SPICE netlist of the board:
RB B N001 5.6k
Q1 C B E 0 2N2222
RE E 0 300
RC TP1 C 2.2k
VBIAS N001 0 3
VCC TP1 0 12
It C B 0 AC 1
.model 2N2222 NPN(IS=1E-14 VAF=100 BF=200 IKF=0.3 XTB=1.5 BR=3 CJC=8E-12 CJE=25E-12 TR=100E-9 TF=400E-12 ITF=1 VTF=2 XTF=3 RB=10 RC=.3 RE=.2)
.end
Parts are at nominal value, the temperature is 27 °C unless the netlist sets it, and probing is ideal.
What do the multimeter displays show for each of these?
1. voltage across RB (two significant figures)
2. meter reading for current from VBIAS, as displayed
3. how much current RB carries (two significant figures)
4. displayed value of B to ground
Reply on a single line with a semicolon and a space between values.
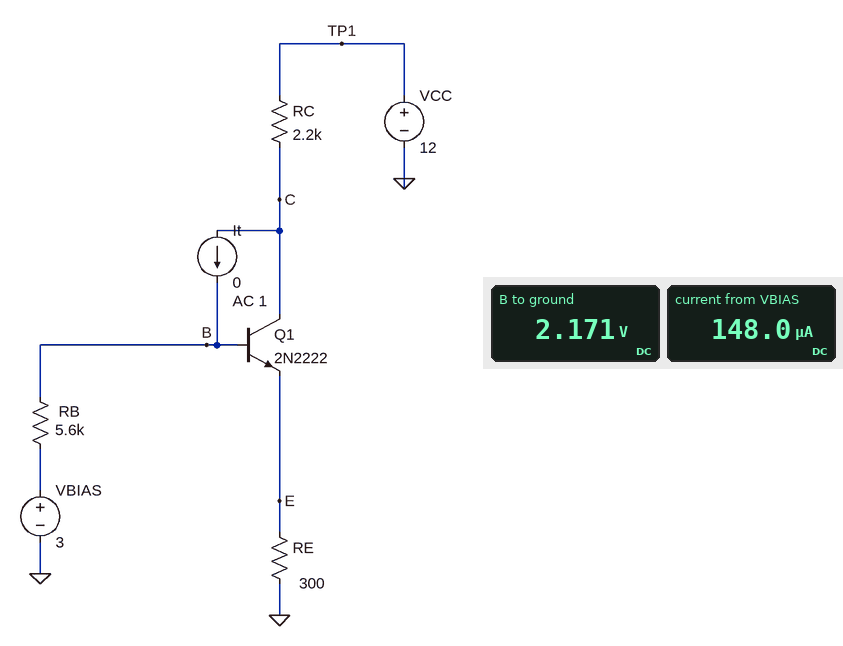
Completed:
830 mV; 148.0 µA; 150 µA; 2.171 V
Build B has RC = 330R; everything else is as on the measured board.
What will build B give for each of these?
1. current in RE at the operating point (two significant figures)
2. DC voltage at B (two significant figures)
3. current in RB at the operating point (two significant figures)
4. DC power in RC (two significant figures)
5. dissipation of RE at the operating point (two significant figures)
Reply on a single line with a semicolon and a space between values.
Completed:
7.0 mA; 2.8 V; 33 µA; 16 mW; 15 mW
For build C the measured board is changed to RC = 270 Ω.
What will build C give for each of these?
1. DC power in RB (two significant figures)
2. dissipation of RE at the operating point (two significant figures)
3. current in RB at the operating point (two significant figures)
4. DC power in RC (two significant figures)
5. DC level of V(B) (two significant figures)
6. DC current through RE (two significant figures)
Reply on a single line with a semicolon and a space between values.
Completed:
6.2 µW; 15 mW; 33 µA; 13 mW; 2.8 V; 7.0 mA
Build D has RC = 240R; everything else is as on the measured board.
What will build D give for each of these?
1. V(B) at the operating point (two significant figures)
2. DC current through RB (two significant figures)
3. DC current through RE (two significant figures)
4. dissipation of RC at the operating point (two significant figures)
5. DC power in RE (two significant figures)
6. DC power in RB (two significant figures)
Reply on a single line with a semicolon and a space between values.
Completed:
2.8 V; 33 µA; 7.0 mA; 12 mW; 15 mW; 6.2 µW
